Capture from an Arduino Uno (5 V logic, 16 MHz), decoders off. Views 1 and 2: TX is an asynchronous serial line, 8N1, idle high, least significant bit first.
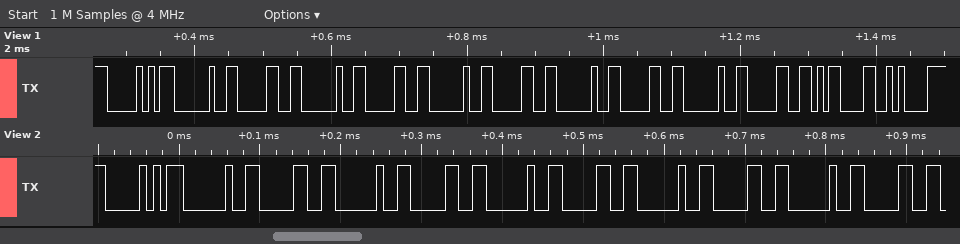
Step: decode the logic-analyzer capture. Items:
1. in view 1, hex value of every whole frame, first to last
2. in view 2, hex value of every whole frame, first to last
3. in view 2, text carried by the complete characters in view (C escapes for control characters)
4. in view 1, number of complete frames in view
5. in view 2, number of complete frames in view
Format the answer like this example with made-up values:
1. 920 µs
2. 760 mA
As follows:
1. 50 20 30 20 30 20 30 20 30 20 30 0D 0A
2. 0x50 0x20 0x30 0x20 0x30 0x20 0x30 0x20 0x30 0x20 0x30
3. "P 0 0 0 0 0"
4. 13
5. 11
